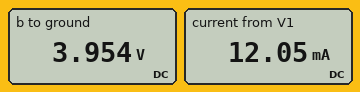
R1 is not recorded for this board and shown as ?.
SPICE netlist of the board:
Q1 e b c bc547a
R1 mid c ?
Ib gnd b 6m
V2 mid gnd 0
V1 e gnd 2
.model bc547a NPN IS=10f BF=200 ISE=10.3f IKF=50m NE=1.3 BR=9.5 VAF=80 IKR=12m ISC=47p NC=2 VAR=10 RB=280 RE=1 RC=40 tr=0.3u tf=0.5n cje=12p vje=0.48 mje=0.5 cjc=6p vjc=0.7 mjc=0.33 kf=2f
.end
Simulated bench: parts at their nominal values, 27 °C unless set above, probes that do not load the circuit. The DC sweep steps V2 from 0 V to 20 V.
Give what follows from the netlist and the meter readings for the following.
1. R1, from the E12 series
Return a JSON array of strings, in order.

["82 Ω"]
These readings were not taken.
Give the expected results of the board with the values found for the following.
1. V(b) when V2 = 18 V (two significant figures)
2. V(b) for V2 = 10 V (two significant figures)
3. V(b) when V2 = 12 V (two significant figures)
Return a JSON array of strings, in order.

["6.3 V", "5.8 V", "5.9 V"]
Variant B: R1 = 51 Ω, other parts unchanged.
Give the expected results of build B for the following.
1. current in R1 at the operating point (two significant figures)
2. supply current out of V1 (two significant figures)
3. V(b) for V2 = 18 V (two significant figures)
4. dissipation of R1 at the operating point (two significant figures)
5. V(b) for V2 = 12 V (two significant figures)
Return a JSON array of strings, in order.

["24 mA", "18 mA", "6.4 V", "30 mW", "6.0 V"]
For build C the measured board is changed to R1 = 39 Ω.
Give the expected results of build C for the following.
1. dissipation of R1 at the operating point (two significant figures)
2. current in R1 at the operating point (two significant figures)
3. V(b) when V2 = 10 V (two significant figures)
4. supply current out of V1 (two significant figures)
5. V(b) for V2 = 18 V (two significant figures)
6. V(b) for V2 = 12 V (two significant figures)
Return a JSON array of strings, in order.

["30 mW", "28 mA", "5.9 V", "22 mA", "6.4 V", "6.0 V"]
